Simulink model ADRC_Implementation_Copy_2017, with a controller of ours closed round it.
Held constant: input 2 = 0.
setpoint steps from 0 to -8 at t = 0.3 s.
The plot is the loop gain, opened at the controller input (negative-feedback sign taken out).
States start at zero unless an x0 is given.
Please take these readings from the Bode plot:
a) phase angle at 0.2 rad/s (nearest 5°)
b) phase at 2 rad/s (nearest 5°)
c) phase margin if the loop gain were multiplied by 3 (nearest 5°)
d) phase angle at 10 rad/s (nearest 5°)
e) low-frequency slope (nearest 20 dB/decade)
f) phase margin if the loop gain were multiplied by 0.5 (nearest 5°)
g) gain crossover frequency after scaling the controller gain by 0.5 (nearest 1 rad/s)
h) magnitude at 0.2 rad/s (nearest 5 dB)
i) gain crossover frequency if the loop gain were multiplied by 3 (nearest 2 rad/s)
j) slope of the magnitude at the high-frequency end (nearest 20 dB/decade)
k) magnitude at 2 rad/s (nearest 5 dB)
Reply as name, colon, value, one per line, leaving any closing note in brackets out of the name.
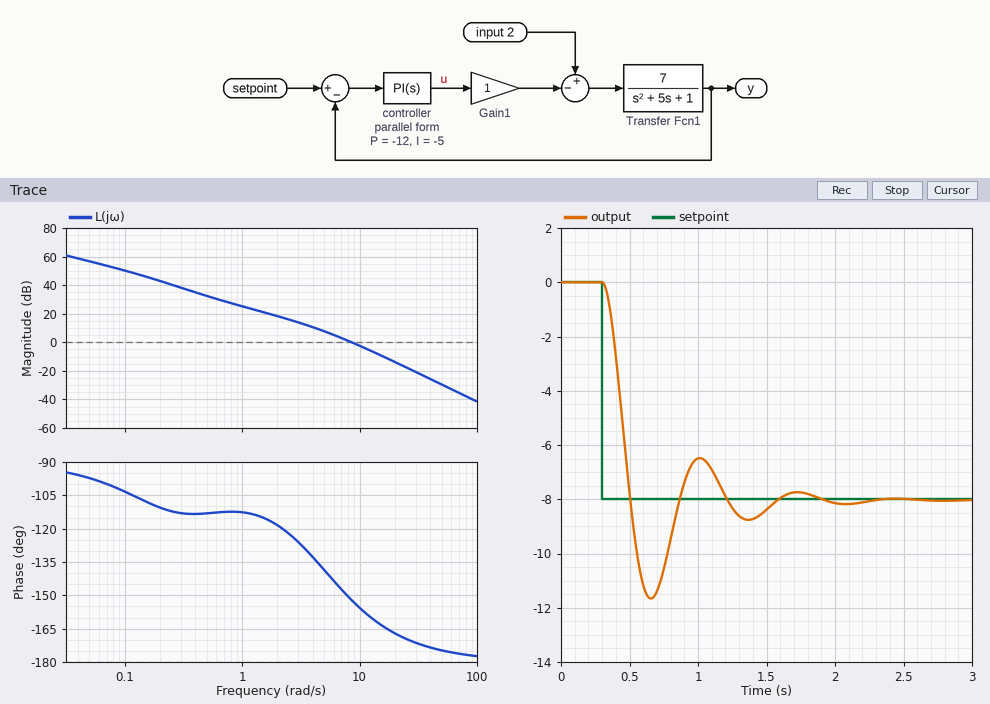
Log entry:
phase angle at 0.2 rad/s: -110°
phase at 2 rad/s: -120°
phase margin if the loop gain were multiplied by 3: 15°
phase angle at 10 rad/s: -155°
low-frequency slope: -20 dB/decade
phase margin if the loop gain were multiplied by 0.5: 40°
gain crossover frequency after scaling the controller gain by 0.5: 6 rad/s
magnitude at 0.2 rad/s: 45 dB
gain crossover frequency if the loop gain were multiplied by 3: 16 rad/s
slope of the magnitude at the high-frequency end: -40 dB/decade
magnitude at 2 rad/s: 20 dB
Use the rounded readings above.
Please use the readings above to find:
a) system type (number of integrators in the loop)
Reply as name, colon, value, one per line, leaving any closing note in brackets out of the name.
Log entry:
system type: 1
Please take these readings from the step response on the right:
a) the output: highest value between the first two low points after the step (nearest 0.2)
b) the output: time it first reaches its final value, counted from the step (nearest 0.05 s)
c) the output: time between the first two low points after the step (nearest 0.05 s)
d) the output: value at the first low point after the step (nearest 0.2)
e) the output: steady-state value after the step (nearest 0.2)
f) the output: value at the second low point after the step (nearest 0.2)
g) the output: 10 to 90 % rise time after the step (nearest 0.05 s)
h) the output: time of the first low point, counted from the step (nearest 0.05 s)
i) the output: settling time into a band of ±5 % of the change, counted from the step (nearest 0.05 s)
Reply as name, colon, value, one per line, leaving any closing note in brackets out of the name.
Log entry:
the output: highest value between the first two low points after the step: -6.4
the output: time it first reaches its final value, counted from the step: 0.20 s
the output: time between the first two low points after the step: 0.70 s
the output: value at the first low point after the step: -11.6
the output: steady-state value after the step: -8.0
the output: value at the second low point after the step: -8.8
the output: 10 to 90 % rise time after the step: 0.15 s
the output: time of the first low point, counted from the step: 0.35 s
the output: settling time into a band of ±5 % of the change, counted from the step: 1.20 s
